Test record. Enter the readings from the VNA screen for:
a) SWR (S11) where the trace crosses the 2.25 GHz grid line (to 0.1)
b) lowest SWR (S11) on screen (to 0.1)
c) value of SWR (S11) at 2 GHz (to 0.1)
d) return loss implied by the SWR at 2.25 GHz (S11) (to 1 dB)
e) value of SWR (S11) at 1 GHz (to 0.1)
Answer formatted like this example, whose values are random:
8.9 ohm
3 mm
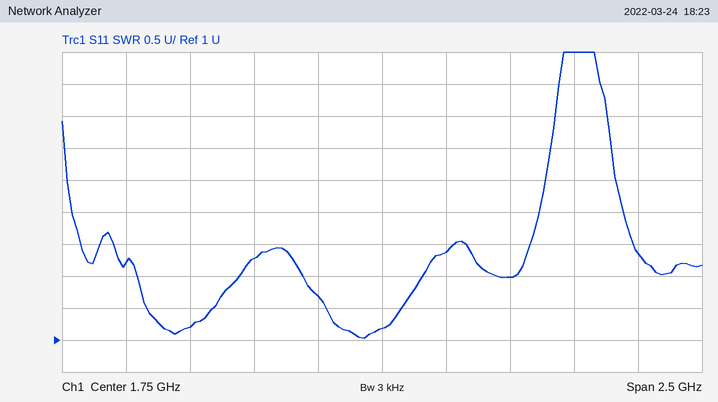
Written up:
2.0
1.0
2.4
10 dB
1.2
